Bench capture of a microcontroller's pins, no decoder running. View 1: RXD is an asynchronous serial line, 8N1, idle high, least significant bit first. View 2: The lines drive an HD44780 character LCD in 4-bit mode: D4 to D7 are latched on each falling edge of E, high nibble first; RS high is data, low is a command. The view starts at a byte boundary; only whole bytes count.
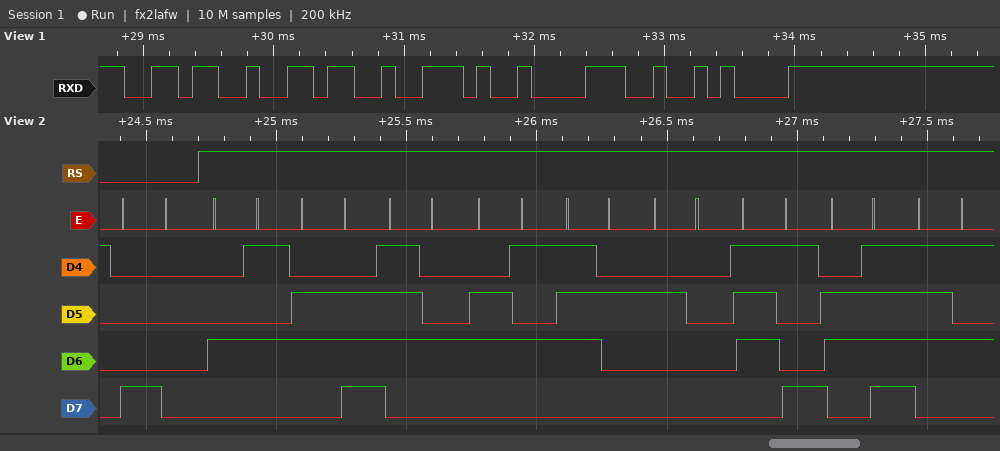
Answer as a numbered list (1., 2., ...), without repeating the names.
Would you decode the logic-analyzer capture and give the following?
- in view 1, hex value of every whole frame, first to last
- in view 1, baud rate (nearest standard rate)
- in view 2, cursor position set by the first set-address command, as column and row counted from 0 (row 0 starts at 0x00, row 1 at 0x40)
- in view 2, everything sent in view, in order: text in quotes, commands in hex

1. 0x36 0x36 0x2E 0x38 0x0A
2. 9600 baud
3. column 0, row 0
4. 0x80 "Enter you"
